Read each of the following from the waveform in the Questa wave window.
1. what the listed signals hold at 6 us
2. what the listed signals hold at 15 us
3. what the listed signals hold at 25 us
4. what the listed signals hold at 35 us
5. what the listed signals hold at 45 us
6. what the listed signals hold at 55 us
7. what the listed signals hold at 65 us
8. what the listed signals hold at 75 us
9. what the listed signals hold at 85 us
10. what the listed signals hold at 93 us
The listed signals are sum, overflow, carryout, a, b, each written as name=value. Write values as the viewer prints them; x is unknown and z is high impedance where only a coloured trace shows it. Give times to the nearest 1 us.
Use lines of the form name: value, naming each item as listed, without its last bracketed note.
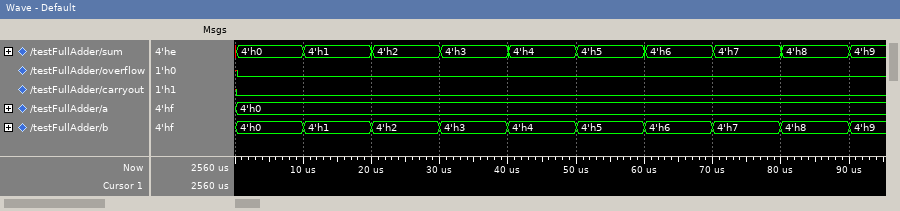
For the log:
what the listed signals hold at 6 us: sum=4'h0, overflow=0, carryout=0, a=4'h0, b=4'h0
what the listed signals hold at 15 us: sum=4'h1, overflow=0, carryout=0, a=4'h0, b=4'h1
what the listed signals hold at 25 us: sum=4'h2, overflow=0, carryout=0, a=4'h0, b=4'h2
what the listed signals hold at 35 us: sum=4'h3, overflow=0, carryout=0, a=4'h0, b=4'h3
what the listed signals hold at 45 us: sum=4'h4, overflow=0, carryout=0, a=4'h0, b=4'h4
what the listed signals hold at 55 us: sum=4'h5, overflow=0, carryout=0, a=4'h0, b=4'h5
what the listed signals hold at 65 us: sum=4'h6, overflow=0, carryout=0, a=4'h0, b=4'h6
what the listed signals hold at 75 us: sum=4'h7, overflow=0, carryout=0, a=4'h0, b=4'h7
what the listed signals hold at 85 us: sum=4'h8, overflow=0, carryout=0, a=4'h0, b=4'h8
what the listed signals hold at 93 us: sum=4'h9, overflow=0, carryout=0, a=4'h0, b=4'h9
